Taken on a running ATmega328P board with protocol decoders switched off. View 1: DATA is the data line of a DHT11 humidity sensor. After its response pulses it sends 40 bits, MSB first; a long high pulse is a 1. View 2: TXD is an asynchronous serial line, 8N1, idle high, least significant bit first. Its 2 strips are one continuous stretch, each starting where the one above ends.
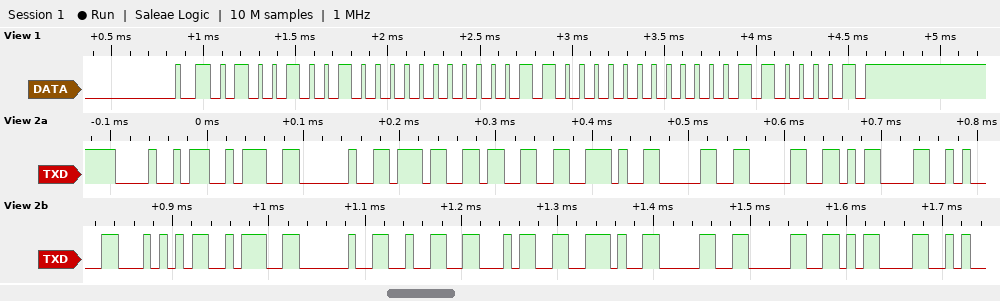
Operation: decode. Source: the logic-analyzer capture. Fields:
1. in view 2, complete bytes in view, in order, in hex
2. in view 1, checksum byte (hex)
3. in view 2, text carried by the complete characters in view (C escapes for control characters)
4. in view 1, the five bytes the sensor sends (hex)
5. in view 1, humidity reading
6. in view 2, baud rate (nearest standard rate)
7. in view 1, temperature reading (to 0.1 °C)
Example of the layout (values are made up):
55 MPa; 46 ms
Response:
0x48 0x3A 0x20 0x37 0x33 0x2E 0x30 0x30 0x0D 0x0A 0x54 0x3A 0x20 0x32 0x34 0x2E 0x30 0x30 0x0D; 0x61; "H: 73.00\r\nT: 24.00\r"; 49 00 18 00 61; 73 %; 115200 baud; 24.0 °C
